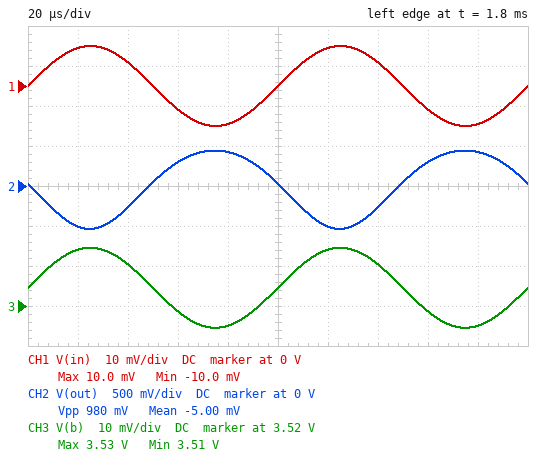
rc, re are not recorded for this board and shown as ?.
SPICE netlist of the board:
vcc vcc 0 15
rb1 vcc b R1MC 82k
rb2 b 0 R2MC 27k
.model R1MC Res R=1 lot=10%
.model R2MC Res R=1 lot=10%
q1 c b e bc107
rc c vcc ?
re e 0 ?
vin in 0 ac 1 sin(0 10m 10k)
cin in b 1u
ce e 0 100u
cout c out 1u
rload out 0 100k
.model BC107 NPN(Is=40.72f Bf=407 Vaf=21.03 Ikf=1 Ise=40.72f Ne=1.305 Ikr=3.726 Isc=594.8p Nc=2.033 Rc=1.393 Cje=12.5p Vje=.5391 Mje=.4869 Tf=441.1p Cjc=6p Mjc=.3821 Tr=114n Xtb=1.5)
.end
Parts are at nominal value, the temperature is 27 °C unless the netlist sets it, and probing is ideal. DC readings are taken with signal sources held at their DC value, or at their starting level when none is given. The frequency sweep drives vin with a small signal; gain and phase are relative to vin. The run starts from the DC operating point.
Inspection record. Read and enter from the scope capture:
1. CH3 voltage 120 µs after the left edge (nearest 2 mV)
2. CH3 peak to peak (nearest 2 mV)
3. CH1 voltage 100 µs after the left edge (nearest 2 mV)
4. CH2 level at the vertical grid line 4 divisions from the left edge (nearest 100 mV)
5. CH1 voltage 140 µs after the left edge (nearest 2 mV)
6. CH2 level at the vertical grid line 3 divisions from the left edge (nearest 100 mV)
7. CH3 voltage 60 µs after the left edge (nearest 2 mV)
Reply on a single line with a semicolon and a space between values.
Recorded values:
3.534 V; 20 mV; 0 V; 400 mV; 6 mV; 300 mV; 3.518 V
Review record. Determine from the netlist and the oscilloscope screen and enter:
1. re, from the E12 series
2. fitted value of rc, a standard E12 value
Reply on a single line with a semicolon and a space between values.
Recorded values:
1.2 kΩ; 560 Ω
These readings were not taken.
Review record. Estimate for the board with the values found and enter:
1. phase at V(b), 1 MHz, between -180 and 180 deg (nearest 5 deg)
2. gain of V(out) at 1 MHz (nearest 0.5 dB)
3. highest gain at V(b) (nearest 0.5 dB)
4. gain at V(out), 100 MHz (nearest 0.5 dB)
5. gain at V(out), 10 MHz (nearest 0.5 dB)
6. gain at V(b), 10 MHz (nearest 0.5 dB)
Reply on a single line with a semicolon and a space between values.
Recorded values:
0 deg; 34.0 dB; 0 dB; 32.0 dB; 34.0 dB; 0 dB
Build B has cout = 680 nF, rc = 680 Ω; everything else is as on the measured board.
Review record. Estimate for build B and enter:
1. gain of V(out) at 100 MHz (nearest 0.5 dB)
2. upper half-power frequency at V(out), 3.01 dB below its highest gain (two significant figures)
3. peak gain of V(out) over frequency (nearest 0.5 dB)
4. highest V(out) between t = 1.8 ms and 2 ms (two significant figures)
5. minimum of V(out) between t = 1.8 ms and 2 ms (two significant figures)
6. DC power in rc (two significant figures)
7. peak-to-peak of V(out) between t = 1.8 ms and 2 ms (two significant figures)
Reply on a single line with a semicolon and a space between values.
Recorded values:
33.0 dB; 110 MHz; 35.5 dB; 530 mV; -640 mV; 3.9 mW; 1.2 V
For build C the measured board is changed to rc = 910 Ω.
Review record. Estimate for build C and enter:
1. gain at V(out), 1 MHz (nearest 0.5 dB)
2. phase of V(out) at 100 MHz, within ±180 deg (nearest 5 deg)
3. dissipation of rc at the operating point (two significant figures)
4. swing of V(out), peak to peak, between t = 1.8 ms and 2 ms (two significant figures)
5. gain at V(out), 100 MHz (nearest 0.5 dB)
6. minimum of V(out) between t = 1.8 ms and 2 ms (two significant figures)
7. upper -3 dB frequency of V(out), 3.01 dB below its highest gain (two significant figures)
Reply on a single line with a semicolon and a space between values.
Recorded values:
38.0 dB; 130 deg; 5.2 mW; 1.5 V; 34.0 dB; -840 mV; 85 MHz
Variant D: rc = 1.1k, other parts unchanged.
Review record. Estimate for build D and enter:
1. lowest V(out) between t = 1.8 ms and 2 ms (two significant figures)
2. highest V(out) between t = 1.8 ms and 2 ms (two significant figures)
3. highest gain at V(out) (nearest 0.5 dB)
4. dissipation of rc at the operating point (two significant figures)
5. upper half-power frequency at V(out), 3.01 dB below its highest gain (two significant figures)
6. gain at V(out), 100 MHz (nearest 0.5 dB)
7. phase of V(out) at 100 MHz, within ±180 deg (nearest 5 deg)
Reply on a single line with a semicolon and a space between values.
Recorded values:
-990 mV; 840 mV; 39.5 dB; 6.3 mW; 70 MHz; 34.5 dB; 125 deg
